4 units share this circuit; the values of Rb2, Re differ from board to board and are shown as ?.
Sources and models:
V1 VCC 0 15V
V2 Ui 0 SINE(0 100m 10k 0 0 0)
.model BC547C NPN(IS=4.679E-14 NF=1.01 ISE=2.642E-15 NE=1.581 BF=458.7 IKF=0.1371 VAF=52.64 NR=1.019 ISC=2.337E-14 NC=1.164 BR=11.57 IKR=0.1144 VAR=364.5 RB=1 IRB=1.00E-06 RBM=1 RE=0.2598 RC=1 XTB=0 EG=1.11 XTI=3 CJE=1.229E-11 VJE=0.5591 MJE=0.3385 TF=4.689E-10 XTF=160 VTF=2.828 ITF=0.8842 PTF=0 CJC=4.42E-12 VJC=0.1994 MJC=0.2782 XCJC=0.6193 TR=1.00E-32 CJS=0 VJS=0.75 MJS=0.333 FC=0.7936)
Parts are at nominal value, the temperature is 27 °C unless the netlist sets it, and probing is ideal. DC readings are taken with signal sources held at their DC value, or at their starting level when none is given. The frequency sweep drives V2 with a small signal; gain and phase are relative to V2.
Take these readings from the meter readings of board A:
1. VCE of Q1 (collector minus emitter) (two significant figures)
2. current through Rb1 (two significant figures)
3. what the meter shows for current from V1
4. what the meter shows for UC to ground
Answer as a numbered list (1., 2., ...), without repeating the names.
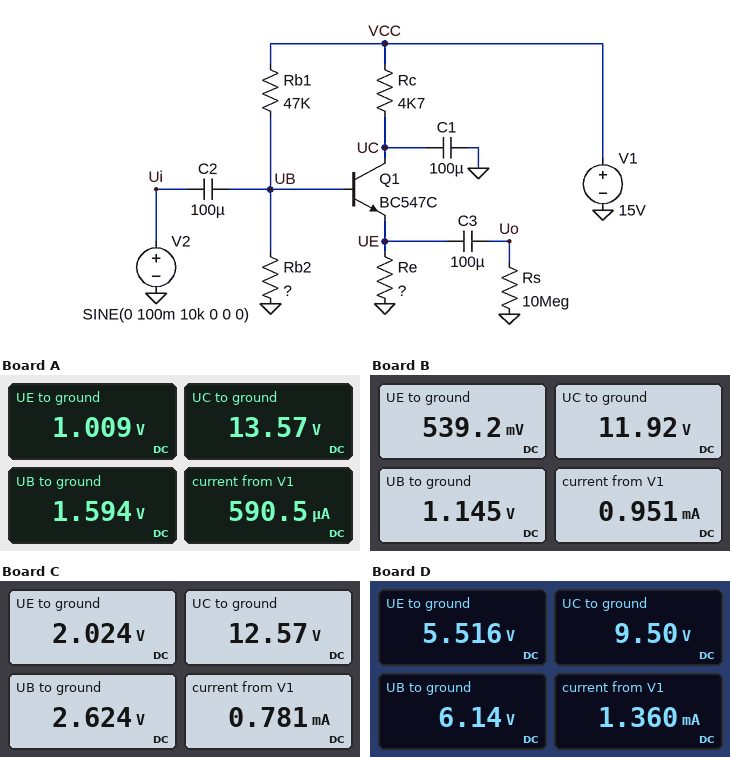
1. 13 V
2. 290 µA
3. 590.5 µA
4. 13.57 V
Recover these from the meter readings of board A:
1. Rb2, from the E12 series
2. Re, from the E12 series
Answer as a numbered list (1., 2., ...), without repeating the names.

1. 5.6 kΩ
2. 3.3 kΩ
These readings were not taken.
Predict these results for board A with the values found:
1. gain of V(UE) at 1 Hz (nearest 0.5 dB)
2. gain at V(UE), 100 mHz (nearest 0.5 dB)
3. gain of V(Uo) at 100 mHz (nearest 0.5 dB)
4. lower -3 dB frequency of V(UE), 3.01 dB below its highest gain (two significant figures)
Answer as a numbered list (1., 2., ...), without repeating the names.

1. -0.5 dB
2. -10.5 dB
3. -10.5 dB
4. 320 mHz
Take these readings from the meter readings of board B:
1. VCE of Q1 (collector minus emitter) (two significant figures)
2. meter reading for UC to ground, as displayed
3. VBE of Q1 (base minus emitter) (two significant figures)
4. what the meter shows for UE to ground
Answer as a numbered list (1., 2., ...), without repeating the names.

1. 11 V
2. 11.92 V
3. 610 mV
4. 539.2 mV
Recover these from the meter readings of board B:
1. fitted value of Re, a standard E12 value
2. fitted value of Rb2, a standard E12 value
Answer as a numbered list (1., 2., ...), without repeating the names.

1. 820 Ω
2. 3.9 kΩ
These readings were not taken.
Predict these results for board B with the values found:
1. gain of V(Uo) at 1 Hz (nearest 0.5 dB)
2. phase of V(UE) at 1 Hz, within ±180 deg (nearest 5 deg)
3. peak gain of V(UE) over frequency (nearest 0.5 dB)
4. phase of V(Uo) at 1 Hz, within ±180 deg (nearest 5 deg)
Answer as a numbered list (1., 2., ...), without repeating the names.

1. -1.0 dB
2. 25 deg
3. -0.5 dB
4. 25 deg
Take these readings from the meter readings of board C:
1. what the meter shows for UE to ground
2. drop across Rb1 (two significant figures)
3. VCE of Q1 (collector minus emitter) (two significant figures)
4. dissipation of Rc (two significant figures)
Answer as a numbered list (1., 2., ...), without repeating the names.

1. 2.024 V
2. 12 V
3. 11 V
4. 1.3 mW
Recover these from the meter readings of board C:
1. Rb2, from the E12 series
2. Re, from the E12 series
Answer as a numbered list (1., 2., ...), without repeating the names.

1. 10 kΩ
2. 3.9 kΩ
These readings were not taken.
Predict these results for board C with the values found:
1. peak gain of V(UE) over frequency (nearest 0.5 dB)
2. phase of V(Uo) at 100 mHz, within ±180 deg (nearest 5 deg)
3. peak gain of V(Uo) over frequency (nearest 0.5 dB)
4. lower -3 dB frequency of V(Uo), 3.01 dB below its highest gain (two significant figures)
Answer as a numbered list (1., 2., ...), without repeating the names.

1. 0 dB
2. 65 deg
3. 0 dB
4. 190 mHz
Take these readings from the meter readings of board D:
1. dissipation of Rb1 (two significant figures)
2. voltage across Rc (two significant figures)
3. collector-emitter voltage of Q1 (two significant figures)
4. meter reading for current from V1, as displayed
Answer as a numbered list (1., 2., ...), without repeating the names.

1. 1.7 mW
2. 5.5 V
3. 4.0 V
4. 1.360 mA
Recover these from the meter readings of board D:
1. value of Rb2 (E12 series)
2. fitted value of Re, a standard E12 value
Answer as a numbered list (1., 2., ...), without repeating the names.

1. 33 kΩ
2. 4.7 kΩ
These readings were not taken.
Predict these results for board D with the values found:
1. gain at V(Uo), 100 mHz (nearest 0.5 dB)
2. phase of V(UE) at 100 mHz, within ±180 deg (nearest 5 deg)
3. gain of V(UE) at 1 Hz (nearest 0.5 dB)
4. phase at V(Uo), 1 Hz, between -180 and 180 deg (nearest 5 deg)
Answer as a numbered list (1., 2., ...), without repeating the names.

1. -2.5 dB
2. 40 deg
3. 0 dB
4. 5 deg
